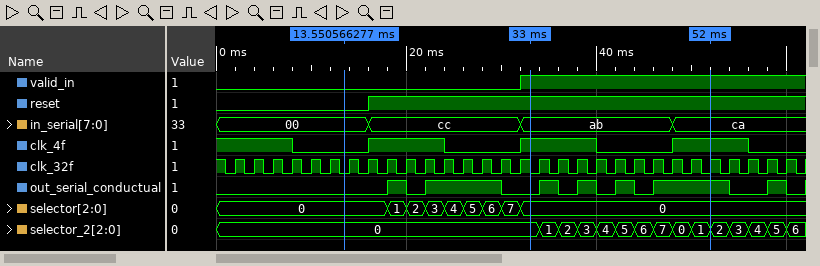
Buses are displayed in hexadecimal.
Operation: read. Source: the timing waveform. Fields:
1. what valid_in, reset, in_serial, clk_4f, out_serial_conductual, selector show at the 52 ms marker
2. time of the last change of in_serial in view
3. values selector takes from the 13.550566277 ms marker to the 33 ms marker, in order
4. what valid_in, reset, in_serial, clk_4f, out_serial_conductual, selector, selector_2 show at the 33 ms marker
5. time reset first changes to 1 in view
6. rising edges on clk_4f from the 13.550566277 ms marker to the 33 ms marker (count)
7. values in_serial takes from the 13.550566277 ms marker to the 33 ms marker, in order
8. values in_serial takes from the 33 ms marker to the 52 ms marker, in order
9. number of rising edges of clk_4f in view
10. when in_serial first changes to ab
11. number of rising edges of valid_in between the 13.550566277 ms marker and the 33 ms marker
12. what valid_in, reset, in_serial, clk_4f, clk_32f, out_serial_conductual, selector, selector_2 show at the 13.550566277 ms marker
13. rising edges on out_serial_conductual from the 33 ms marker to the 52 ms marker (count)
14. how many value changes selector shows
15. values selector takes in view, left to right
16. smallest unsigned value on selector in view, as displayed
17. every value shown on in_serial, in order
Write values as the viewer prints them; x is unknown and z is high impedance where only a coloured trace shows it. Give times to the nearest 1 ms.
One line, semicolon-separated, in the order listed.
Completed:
valid_in=1, reset=1, in_serial=ca, clk_4f=1, out_serial_conductual=1, selector=0; 48 ms; 0, 1, 2, 3, 4, 5, 6, 7, 0; valid_in=1, reset=1, in_serial=ab, clk_4f=1, out_serial_conductual=0, selector=0, selector_2=0; 16 ms; 2; 00, cc, ab; ab, ca; 3; 32 ms; 1; valid_in=0, reset=0, in_serial=00, clk_4f=0, clk_32f=0, out_serial_conductual=0, selector=0, selector_2=0; 4; 8; 0, 1, 2, 3, 4, 5, 6, 7, 0; 0; 00, cc, ab, ca
